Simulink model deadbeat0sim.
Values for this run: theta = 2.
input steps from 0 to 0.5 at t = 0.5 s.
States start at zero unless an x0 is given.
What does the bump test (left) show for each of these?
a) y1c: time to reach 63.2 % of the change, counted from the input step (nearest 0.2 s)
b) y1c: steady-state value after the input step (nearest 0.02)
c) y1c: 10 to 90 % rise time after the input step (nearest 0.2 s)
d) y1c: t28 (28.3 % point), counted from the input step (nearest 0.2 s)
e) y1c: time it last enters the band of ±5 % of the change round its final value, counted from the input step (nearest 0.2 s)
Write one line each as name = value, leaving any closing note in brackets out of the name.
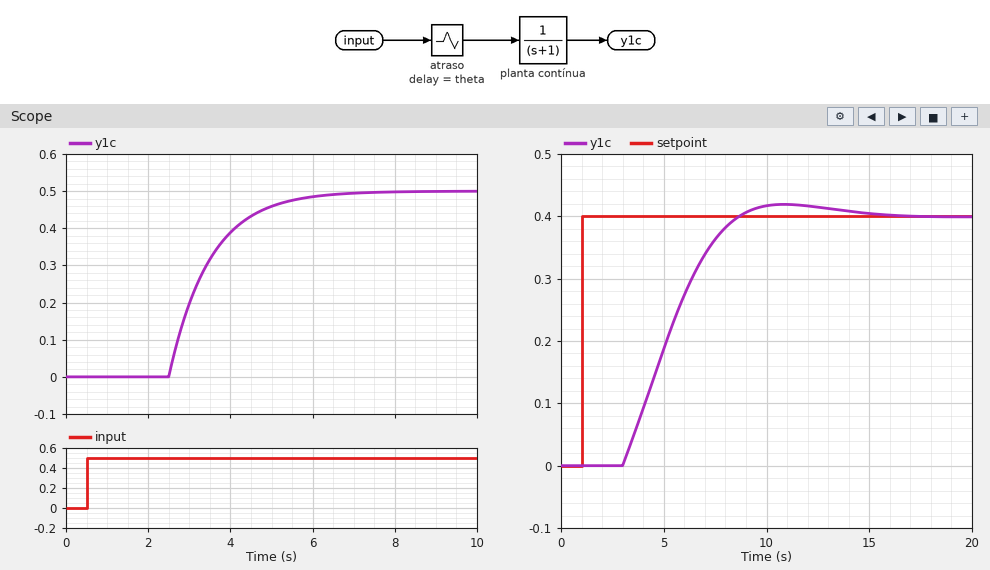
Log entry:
y1c: time to reach 63.2 % of the change, counted from the input step = 3.0 s
y1c: steady-state value after the input step = 0.50
y1c: 10 to 90 % rise time after the input step = 2.2 s
y1c: t28 (28.3 % point), counted from the input step = 2.4 s
y1c: time it last enters the band of ±5 % of the change round its final value, counted from the input step = 5.0 s
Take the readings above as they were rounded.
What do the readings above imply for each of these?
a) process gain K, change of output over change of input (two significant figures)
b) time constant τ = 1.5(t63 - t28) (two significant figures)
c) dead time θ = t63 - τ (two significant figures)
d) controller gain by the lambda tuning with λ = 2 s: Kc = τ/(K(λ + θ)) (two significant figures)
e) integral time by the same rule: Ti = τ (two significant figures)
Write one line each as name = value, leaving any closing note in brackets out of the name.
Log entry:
process gain K, change of output over change of input = 1.0
time constant τ = 1.5(t63 - t28) = 0.90 s
dead time θ = t63 - τ = 2.1 s
controller gain by the lambda tuning with λ = 2 s: Kc = τ/(K(λ + θ)) = 0.22
integral time by the same rule: Ti = τ = 0.90 s
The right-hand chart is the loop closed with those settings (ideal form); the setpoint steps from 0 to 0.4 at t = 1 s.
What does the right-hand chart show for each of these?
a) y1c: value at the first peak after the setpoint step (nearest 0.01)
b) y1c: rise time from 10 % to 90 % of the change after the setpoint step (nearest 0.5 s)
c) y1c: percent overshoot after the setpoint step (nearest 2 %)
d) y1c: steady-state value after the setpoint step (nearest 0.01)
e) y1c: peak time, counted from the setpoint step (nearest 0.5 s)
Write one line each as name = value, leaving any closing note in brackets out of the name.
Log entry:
y1c: value at the first peak after the setpoint step = 0.42
y1c: rise time from 10 % to 90 % of the change after the setpoint step = 4.0 s
y1c: percent overshoot after the setpoint step = 4 %
y1c: steady-state value after the setpoint step = 0.40
y1c: peak time, counted from the setpoint step = 10.0 s
